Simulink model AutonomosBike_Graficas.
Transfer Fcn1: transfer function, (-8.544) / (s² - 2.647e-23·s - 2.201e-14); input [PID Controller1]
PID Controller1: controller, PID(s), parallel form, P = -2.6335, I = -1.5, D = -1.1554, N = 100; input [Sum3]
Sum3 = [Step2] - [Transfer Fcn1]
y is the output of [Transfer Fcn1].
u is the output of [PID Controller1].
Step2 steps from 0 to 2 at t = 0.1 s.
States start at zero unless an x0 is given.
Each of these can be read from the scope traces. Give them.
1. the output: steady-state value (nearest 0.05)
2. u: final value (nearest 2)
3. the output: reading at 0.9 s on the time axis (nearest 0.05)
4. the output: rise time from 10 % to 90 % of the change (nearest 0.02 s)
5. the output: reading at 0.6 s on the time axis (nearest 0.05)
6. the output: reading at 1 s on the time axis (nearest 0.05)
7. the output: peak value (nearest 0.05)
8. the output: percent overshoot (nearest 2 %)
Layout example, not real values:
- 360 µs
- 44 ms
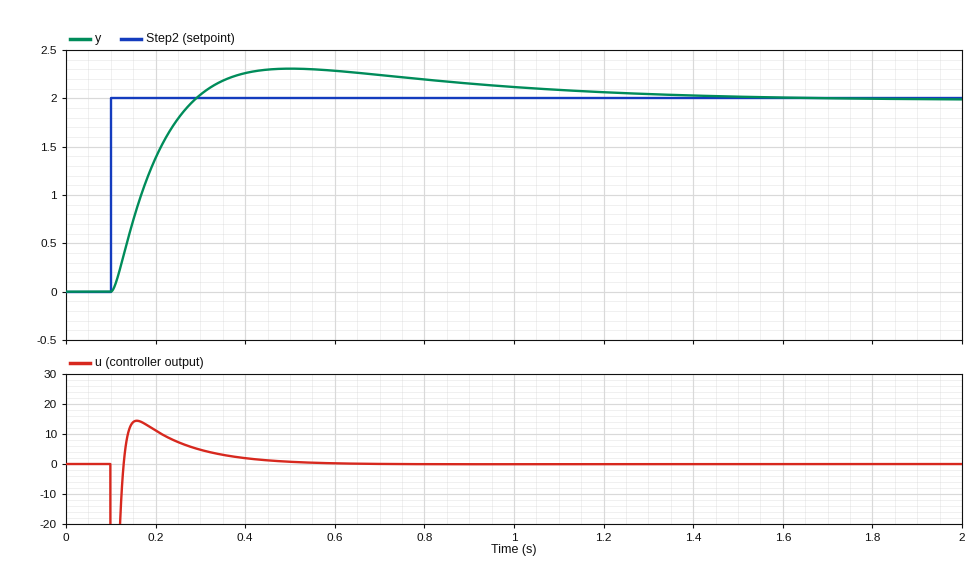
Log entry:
- 2.00
- 0
- 2.15
- 0.14 s
- 2.30
- 2.10
- 2.30
- 16 %
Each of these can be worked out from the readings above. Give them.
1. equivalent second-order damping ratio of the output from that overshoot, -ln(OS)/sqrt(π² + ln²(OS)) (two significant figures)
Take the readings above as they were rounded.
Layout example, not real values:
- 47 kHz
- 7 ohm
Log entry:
- 0.50
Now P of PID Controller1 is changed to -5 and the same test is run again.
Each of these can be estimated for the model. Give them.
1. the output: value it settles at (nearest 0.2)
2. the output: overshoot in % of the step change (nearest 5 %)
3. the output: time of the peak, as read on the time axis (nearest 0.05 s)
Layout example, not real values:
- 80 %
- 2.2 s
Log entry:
- 2.0
- 20 %
- 0.40 s
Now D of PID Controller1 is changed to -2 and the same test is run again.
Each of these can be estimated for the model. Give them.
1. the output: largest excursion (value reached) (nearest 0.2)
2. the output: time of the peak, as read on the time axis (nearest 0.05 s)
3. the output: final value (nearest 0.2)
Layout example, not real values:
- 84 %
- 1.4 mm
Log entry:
- 2.2
- 0.40 s
- 2.0
